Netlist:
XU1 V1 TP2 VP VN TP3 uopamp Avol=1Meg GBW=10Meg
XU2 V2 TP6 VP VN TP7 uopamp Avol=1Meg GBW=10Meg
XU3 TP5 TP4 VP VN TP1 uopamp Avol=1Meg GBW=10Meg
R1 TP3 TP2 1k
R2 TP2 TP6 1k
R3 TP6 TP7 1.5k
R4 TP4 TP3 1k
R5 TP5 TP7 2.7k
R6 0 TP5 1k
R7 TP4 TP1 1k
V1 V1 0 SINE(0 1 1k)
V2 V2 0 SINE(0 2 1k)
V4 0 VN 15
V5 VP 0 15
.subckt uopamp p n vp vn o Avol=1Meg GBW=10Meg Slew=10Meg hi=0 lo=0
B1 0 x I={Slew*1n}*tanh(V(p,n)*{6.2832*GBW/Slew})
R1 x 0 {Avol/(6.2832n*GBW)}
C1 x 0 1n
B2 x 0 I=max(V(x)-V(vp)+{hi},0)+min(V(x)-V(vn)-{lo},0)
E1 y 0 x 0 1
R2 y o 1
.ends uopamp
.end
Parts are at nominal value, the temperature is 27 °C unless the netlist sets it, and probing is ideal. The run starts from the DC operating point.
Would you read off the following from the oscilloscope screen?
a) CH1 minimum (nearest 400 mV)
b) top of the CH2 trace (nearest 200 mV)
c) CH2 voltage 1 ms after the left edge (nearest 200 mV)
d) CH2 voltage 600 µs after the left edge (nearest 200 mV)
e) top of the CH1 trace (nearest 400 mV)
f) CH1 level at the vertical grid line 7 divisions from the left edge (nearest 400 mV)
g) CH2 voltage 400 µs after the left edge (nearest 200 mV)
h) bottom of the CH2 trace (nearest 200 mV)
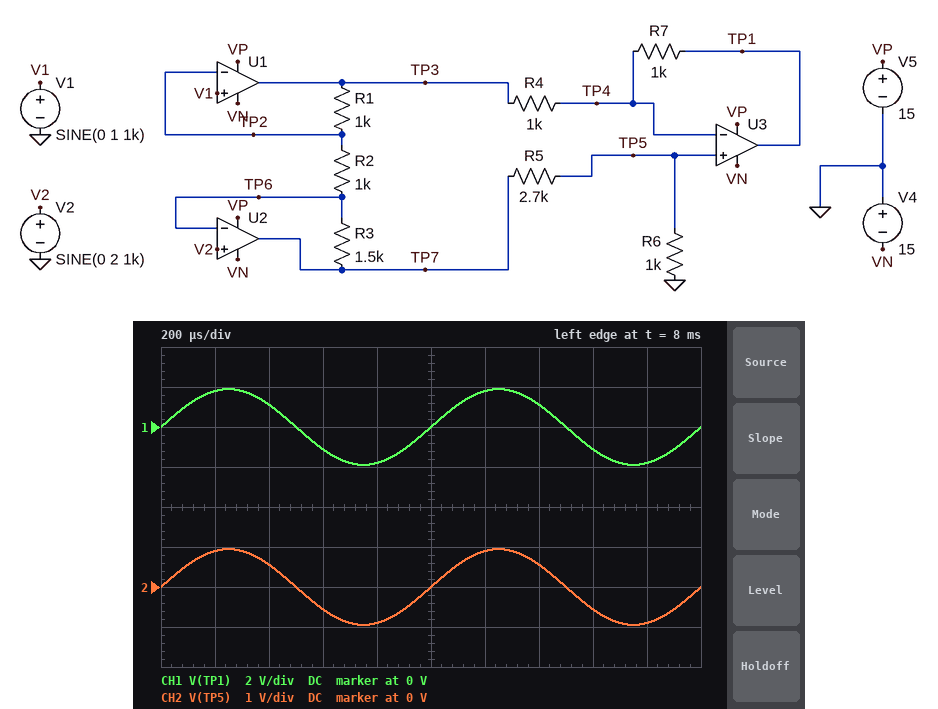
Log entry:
-2.0 V
1.0 V
0 V
-600 mV
2.0 V
1.2 V
600 mV
-1.0 V
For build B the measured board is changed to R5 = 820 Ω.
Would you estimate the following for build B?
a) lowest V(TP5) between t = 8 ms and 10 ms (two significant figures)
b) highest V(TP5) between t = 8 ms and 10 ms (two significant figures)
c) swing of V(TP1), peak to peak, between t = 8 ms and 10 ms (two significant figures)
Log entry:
-1.9 V
1.9 V
7.7 V
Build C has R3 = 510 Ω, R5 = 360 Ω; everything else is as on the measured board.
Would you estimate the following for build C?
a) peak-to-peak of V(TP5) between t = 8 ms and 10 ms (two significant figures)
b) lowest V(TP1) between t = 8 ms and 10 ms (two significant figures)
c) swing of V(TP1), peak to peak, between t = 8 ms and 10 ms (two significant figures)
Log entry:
3.7 V
-3.7 V
7.4 V
